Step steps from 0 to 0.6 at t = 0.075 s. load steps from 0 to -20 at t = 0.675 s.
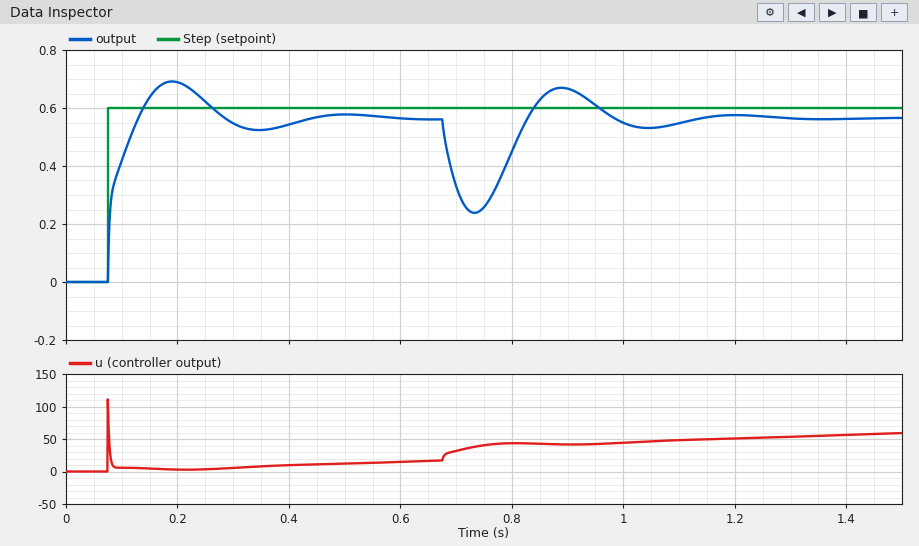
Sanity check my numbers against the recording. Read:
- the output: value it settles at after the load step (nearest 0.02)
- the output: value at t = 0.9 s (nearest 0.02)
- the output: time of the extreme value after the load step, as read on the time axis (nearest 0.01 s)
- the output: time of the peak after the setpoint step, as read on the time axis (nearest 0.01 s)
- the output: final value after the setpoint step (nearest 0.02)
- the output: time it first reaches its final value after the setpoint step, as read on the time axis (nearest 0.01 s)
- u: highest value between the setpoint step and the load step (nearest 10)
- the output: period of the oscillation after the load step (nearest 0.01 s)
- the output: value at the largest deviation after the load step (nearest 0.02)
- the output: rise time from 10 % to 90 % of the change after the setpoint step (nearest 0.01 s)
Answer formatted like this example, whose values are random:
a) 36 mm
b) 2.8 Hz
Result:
a) 0.56
b) 0.66
c) 0.73 s
d) 0.19 s
e) 0.56
f) 0.13 s
g) 110
h) 0.31 s
i) 0.24
j) 0.04 s
